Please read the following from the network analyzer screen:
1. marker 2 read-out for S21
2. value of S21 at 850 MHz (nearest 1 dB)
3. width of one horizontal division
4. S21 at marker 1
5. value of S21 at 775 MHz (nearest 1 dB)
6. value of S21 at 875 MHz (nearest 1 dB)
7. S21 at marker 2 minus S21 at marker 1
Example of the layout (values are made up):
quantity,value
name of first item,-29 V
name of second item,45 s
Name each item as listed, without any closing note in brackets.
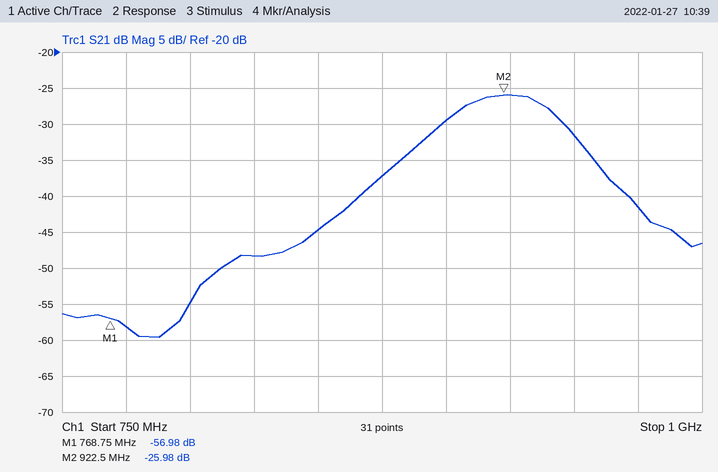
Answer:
quantity,value
marker 2 read-out for S21,-25.98 dB
value of S21 at 850 MHz,-45 dB
width of one horizontal division,25 MHz
S21 at marker 1,-56.98 dB
value of S21 at 775 MHz,-58 dB
value of S21 at 875 MHz,-37 dB
S21 at marker 2 minus S21 at marker 1,31.00 dB
